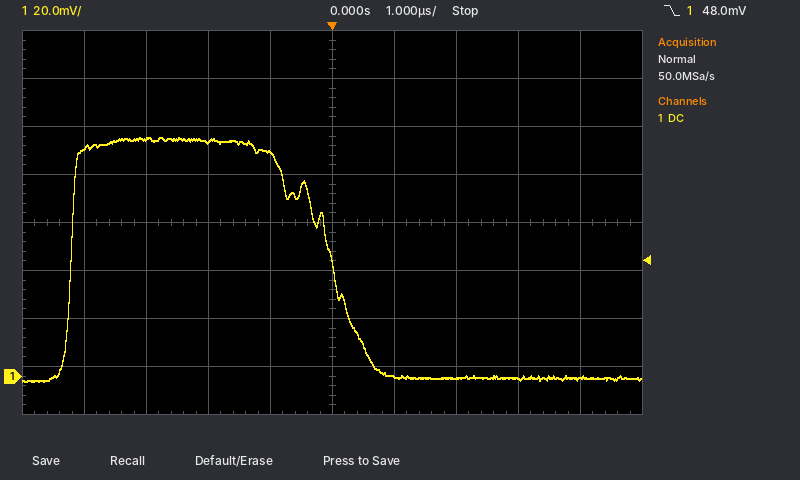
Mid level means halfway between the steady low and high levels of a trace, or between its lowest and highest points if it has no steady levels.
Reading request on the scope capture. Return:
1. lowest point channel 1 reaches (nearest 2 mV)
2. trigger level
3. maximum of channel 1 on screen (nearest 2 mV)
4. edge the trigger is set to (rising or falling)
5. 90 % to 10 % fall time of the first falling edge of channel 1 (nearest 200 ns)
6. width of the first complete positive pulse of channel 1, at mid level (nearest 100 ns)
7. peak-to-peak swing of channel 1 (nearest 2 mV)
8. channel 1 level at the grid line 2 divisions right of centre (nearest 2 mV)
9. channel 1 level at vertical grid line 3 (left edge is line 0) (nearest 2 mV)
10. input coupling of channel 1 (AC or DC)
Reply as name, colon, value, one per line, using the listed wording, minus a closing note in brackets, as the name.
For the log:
lowest point channel 1 reaches: -2 mV
trigger level: 48.0 mV
maximum of channel 1 on screen: 100 mV
edge the trigger is set to: falling
90 % to 10 % fall time of the first falling edge of channel 1: 1.4 µs
width of the first complete positive pulse of channel 1, at mid level: 4.2 µs
peak-to-peak swing of channel 1: 102 mV
channel 1 level at the grid line 2 divisions right of centre: 0 mV
channel 1 level at vertical grid line 3 (left edge is line 0): 98 mV
input coupling of channel 1: DC
